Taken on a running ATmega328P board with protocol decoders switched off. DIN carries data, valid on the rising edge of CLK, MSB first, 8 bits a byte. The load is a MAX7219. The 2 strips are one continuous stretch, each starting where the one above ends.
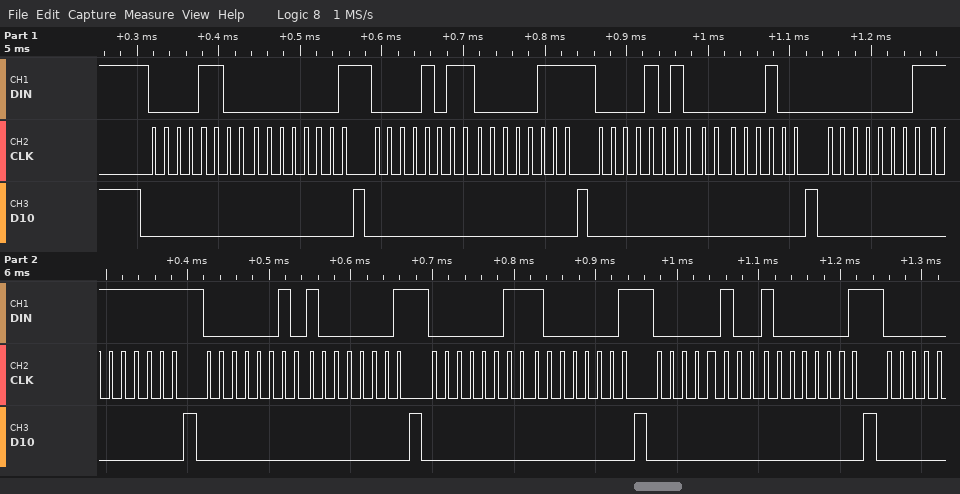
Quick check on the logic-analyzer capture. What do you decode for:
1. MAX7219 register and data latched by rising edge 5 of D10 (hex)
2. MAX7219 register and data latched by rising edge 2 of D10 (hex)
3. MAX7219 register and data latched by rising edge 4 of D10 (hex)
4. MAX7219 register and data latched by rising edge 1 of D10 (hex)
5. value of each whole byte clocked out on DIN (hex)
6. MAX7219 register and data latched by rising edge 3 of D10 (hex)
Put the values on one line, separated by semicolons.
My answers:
register 0x2, data 0x81; register 0xB, data 0x07; register 0x1, data 0xFF; register 0xC, data 0x01; 0C 01 0B 07 0A 04 01 FF 02 81 03 81 04 81; register 0xA, data 0x04
